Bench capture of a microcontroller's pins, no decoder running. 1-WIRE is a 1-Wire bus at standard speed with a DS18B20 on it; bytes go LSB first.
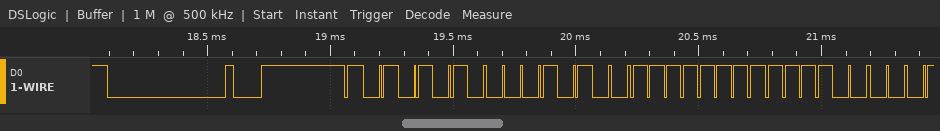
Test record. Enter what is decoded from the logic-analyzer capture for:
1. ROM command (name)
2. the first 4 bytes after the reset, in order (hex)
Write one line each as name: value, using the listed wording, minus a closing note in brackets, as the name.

ROM command: Match ROM
the first 4 bytes after the reset, in order: 55 28 FF 0F
